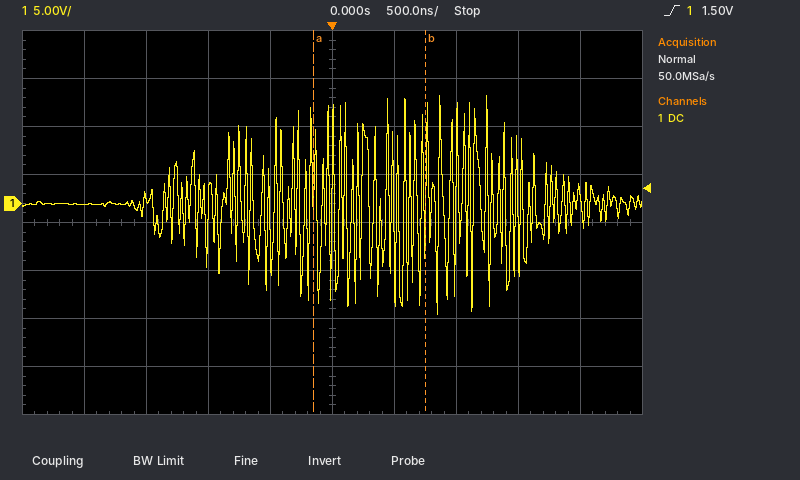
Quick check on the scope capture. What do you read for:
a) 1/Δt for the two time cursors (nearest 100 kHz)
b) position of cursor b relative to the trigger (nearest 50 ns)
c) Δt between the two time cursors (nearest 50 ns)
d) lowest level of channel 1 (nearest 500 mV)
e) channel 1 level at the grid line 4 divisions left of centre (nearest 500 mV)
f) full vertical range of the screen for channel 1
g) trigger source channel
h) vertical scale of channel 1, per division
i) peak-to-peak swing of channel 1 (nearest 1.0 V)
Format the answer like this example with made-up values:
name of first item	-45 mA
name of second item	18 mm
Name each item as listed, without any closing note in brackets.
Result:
1/Δt for the two time cursors	1.1 MHz
position of cursor b relative to the trigger	+750 ns
Δt between the two time cursors	900 ns
lowest level of channel 1	-11.5 V
channel 1 level at the grid line 4 divisions left of centre	0.0 V
full vertical range of the screen for channel 1	40 V
trigger source channel	channel 1
vertical scale of channel 1, per division	5 V
peak-to-peak swing of channel 1	23.0 V
